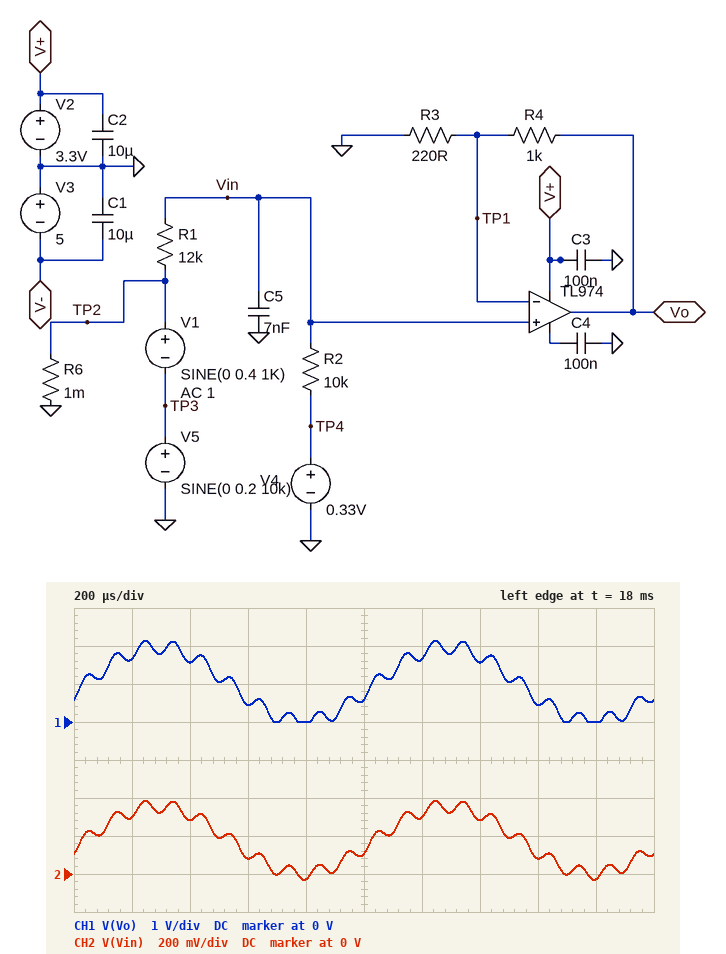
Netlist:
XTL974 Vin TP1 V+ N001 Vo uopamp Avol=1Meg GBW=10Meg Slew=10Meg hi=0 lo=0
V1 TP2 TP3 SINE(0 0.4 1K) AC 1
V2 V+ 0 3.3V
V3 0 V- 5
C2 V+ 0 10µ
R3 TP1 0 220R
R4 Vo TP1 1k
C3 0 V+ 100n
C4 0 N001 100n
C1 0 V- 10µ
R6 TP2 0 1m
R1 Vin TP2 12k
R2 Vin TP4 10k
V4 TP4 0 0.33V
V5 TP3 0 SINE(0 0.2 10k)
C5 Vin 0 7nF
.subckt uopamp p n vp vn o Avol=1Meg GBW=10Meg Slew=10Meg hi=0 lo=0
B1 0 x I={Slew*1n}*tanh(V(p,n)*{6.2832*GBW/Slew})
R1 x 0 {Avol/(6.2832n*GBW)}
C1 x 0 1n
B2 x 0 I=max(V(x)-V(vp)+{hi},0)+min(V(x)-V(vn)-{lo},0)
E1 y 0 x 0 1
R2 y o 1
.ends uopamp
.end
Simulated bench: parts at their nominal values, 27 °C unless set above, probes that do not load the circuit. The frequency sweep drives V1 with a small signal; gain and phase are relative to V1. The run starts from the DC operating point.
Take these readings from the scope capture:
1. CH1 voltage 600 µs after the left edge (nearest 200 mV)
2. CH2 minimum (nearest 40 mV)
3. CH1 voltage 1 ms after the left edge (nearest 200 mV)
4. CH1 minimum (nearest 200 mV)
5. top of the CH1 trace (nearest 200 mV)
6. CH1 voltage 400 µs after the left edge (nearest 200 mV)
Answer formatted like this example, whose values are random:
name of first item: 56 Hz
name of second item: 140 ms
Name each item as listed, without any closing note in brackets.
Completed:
CH1 voltage 600 µs after the left edge: 400 mV
CH2 minimum: -40 mV
CH1 voltage 1 ms after the left edge: 600 mV
CH1 minimum: 0 V
top of the CH1 trace: 2.2 V
CH1 voltage 400 µs after the left edge: 1.6 V
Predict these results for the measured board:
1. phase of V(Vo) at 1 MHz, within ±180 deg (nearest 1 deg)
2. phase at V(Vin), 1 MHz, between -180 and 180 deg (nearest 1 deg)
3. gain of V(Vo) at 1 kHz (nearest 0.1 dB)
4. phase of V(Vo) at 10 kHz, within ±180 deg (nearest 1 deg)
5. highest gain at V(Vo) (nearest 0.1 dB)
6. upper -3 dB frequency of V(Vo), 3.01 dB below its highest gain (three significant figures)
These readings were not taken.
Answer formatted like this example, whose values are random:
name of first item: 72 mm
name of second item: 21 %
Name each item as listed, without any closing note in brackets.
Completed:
phase of V(Vo) at 1 MHz, within ±180 deg: -119 deg
phase at V(Vin), 1 MHz, between -180 and 180 deg: -90 deg
gain of V(Vo) at 1 kHz: 7.8 dB
phase of V(Vo) at 10 kHz, within ±180 deg: -68 deg
highest gain at V(Vo): 8.0 dB
upper -3 dB frequency of V(Vo), 3.01 dB below its highest gain: 4.17 kHz
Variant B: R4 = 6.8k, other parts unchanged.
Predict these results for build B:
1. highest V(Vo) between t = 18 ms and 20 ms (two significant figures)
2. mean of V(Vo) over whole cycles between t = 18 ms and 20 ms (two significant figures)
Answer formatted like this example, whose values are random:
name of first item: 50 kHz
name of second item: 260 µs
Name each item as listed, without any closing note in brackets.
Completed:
highest V(Vo) between t = 18 ms and 20 ms: 3.3 V
mean of V(Vo) over whole cycles between t = 18 ms and 20 ms: 2.6 V
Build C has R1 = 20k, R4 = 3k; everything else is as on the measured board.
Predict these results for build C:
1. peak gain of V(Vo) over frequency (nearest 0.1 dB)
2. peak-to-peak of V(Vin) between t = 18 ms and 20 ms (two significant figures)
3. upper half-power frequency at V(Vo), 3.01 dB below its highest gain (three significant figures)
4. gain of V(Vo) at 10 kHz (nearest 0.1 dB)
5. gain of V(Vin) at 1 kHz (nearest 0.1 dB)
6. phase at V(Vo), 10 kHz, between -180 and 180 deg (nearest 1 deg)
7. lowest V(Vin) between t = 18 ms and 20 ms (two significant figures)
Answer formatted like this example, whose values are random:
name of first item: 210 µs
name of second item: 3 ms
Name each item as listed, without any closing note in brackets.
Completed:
peak gain of V(Vo) over frequency: 13.8 dB
peak-to-peak of V(Vin) between t = 18 ms and 20 ms: 290 mV
upper half-power frequency at V(Vo), 3.01 dB below its highest gain: 3.41 kHz
gain of V(Vo) at 10 kHz: 3.9 dB
gain of V(Vin) at 1 kHz: -9.9 dB
phase at V(Vo), 10 kHz, between -180 and 180 deg: -72 deg
lowest V(Vin) between t = 18 ms and 20 ms: 71 mV
